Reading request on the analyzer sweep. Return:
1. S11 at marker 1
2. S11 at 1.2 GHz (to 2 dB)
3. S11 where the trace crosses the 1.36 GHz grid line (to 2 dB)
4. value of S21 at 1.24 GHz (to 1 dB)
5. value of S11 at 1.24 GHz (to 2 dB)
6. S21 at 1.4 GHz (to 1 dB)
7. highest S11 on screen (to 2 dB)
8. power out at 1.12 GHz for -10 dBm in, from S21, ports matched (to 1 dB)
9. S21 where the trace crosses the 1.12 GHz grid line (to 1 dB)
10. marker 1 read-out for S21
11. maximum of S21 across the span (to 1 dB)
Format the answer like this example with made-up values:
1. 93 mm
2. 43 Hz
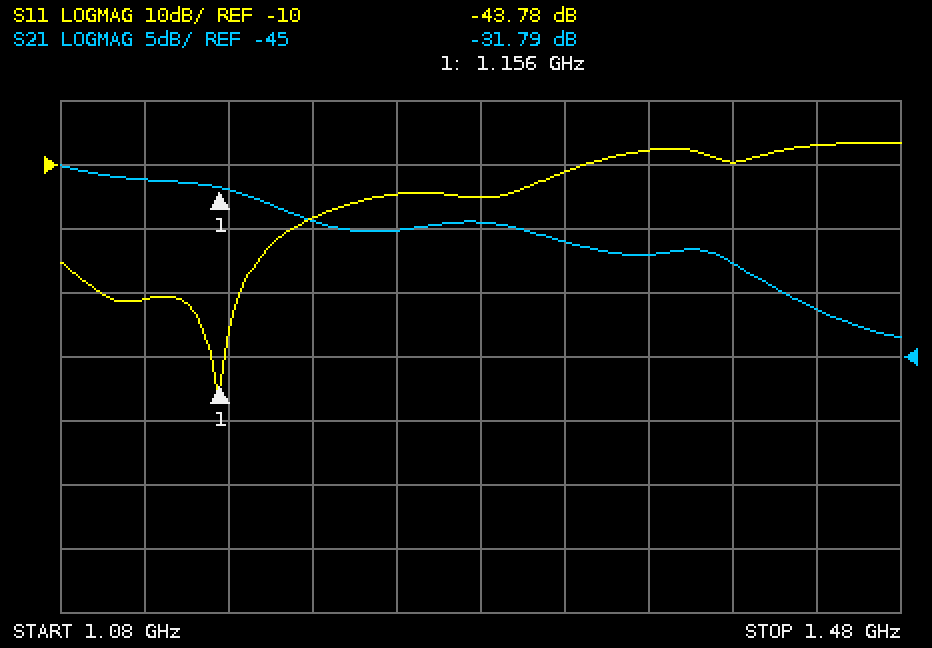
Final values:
1. -43.78 dB
2. -18 dB
3. -8 dB
4. -35 dB
5. -14 dB
6. -38 dB
7. -6 dB
8. -41 dBm
9. -31 dB
10. -31.79 dB
11. -30 dB
